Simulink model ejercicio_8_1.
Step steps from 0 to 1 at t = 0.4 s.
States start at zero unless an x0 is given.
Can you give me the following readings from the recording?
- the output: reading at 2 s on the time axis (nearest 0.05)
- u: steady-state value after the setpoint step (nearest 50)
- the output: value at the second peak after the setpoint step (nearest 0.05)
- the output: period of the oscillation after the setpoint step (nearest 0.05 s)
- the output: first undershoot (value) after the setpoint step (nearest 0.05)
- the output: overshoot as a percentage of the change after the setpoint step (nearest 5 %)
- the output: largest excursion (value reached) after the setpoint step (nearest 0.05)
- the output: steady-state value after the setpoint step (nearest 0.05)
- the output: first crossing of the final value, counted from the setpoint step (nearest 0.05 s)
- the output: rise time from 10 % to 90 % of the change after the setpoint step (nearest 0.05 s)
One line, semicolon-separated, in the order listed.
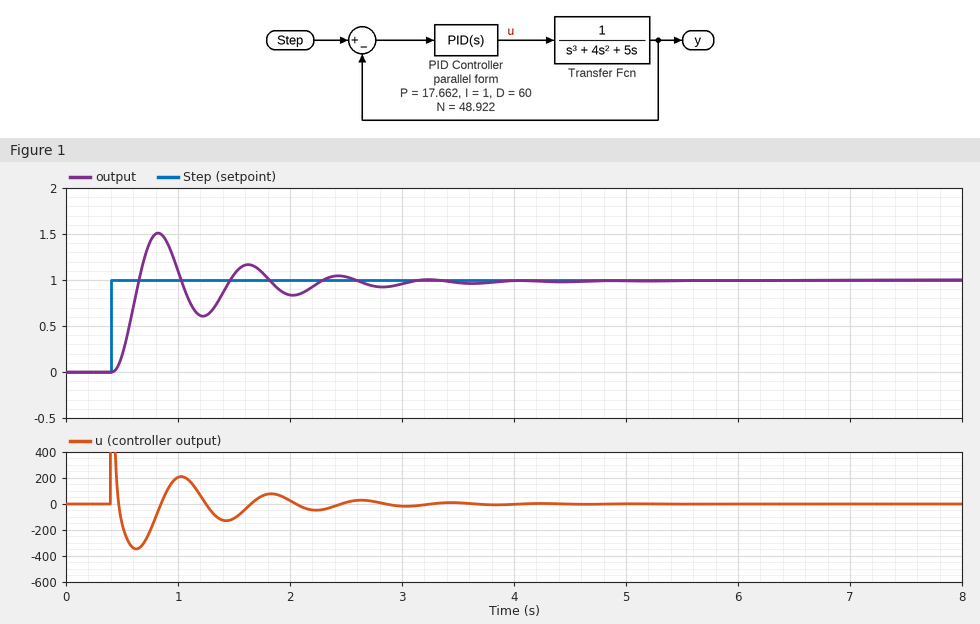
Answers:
0.85; 0; 1.15; 0.80 s; 0.60; 50 %; 1.50; 1.00; 0.25 s; 0.15 s
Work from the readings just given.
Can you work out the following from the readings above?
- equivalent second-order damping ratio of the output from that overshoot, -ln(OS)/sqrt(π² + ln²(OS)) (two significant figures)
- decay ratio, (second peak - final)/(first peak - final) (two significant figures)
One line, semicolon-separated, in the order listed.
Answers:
0.22; 0.30
